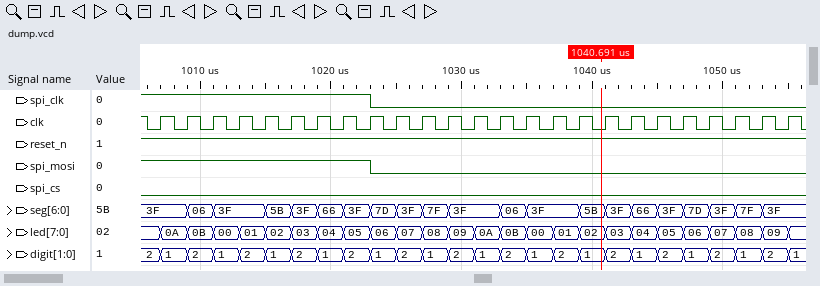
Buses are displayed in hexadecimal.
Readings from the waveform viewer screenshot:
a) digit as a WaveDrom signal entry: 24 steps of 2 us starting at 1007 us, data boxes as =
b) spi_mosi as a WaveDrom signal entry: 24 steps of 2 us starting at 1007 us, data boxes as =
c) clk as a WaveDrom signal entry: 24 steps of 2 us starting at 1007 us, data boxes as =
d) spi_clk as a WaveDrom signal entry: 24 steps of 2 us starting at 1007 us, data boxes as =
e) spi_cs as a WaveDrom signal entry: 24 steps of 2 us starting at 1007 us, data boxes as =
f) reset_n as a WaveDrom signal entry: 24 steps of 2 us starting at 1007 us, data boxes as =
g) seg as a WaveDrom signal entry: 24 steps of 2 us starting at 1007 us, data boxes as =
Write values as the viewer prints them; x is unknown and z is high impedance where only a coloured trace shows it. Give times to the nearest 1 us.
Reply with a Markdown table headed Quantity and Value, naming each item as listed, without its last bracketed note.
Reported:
| Quantity | Value |
|---|---|
| digit as a WaveDrom signal entry: 24 steps of 2 us starting at 1007 us, data boxes as = | {name: 'digit', wave: '========================', data: '1 2 1 2 1 2 1 2 1 2 1 2 1 2 1 2 1 2 1 2 1 2 1 2'} |
| spi_mosi as a WaveDrom signal entry: 24 steps of 2 us starting at 1007 us, data boxes as = | {name: 'spi_mosi', wave: '1.......0...............'} |
| clk as a WaveDrom signal entry: 24 steps of 2 us starting at 1007 us, data boxes as = | {name: 'clk', wave: 'p.......................'} |
| spi_clk as a WaveDrom signal entry: 24 steps of 2 us starting at 1007 us, data boxes as = | {name: 'spi_clk', wave: '1.......0...............'} |
| spi_cs as a WaveDrom signal entry: 24 steps of 2 us starting at 1007 us, data boxes as = | {name: 'spi_cs', wave: '0.......................'} |
| reset_n as a WaveDrom signal entry: 24 steps of 2 us starting at 1007 us, data boxes as = | {name: 'reset_n', wave: '1.......................'} |
| seg as a WaveDrom signal entry: 24 steps of 2 us starting at 1007 us, data boxes as = | {name: 'seg', wave: '===.========.==.========', data: '3F 06 3F 5B 3F 66 3F 7D 3F 7F 3F 06 3F 5B 3F 66 3F 7D 3F 7F 3F'} |
